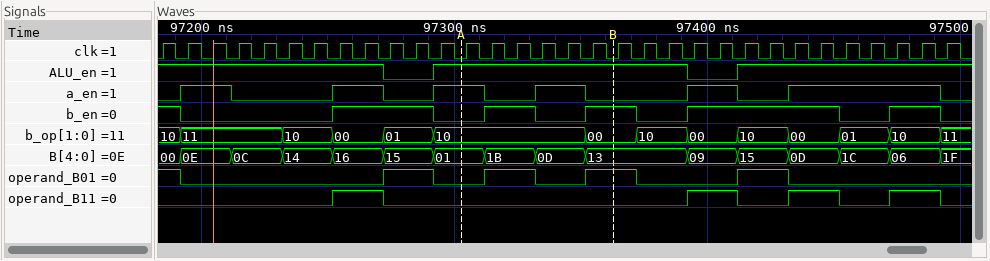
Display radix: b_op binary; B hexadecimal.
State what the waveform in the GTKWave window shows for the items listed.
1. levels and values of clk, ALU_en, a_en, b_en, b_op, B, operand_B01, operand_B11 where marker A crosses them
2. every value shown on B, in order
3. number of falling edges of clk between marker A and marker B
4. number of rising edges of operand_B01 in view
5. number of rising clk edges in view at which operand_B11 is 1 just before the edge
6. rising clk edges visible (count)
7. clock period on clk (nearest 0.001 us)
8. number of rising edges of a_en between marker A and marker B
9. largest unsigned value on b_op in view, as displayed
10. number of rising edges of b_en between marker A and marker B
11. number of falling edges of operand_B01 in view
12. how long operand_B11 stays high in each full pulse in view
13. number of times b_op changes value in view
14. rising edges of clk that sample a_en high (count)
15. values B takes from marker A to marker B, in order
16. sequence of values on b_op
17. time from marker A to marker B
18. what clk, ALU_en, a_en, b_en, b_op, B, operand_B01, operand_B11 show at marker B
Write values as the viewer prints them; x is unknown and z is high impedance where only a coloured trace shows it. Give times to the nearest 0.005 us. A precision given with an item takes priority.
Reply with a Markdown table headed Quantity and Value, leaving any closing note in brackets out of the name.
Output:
| Quantity | Value |
|---|---|
| levels and values of clk, ALU_en, a_en, b_en, b_op, B, operand_B01, operand_B11 where marker A crosses them | clk=0, ALU_en=1, a_en=1, b_en=0, b_op=10, B=01, operand_B01=0, operand_B11=0 |
| every value shown on B, in order | 00, 0E, 0C, 14, 16, 15, 01, 1B, 0D, 13, 09, 15, 0D, 1C, 06, 1F |
| number of falling edges of clk between marker A and marker B | 6 |
| number of rising edges of operand_B01 in view | 4 |
| number of rising clk edges in view at which operand_B11 is 1 just before the edge | 8 |
| rising clk edges visible | 32 |
| clock period on clk | 0.01 us |
| number of rising edges of a_en between marker A and marker B | 1 |
| largest unsigned value on b_op in view, as displayed | 11 |
| number of rising edges of b_en between marker A and marker B | 2 |
| number of falling edges of operand_B01 in view | 5 |
| how long operand_B11 stays high in each full pulse in view | 0.02 us, 0.02 us, 0.02 us, 0.02 us |
| number of times b_op changes value in view | 13 |
| rising edges of clk that sample a_en high | 16 |
| values B takes from marker A to marker B, in order | 01, 1B, 0D, 13 |
| sequence of values on b_op | 10, 11, 10, 00, 01, 10, 00, 10, 00, 10, 00, 01, 10, 11 |
| time from marker A to marker B | 0.06 us |
| what clk, ALU_en, a_en, b_en, b_op, B, operand_B01, operand_B11 show at marker B | clk=0, ALU_en=1, a_en=0, b_en=1, b_op=00, B=13, operand_B01=1, operand_B11=0 |
